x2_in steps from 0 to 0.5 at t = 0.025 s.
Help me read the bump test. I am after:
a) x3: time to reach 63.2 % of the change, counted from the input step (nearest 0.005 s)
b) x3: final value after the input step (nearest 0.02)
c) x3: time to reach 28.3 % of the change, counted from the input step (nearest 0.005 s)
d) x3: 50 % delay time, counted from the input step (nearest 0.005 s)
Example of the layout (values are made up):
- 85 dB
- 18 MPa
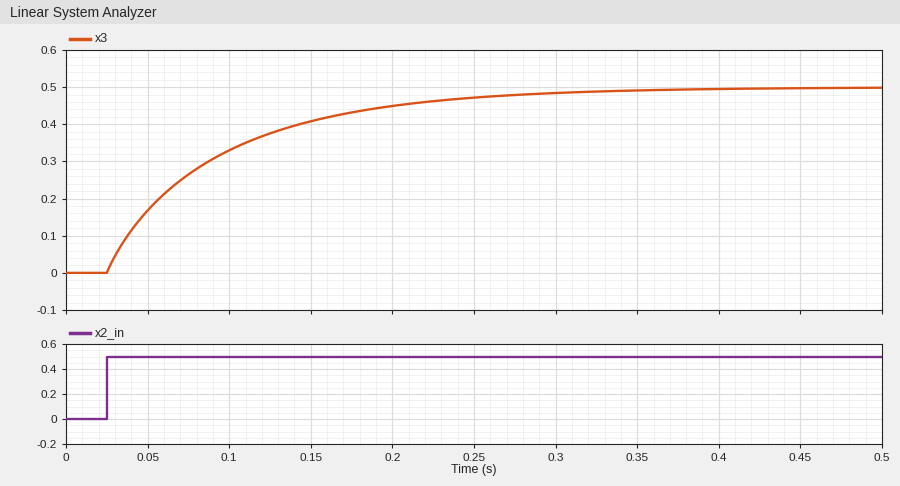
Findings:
- 0.070 s
- 0.50
- 0.020 s
- 0.045 s
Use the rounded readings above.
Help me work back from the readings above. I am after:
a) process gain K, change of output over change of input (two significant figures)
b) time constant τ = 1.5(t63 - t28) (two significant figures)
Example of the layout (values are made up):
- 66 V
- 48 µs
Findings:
- 1.0
- 0.075 s
